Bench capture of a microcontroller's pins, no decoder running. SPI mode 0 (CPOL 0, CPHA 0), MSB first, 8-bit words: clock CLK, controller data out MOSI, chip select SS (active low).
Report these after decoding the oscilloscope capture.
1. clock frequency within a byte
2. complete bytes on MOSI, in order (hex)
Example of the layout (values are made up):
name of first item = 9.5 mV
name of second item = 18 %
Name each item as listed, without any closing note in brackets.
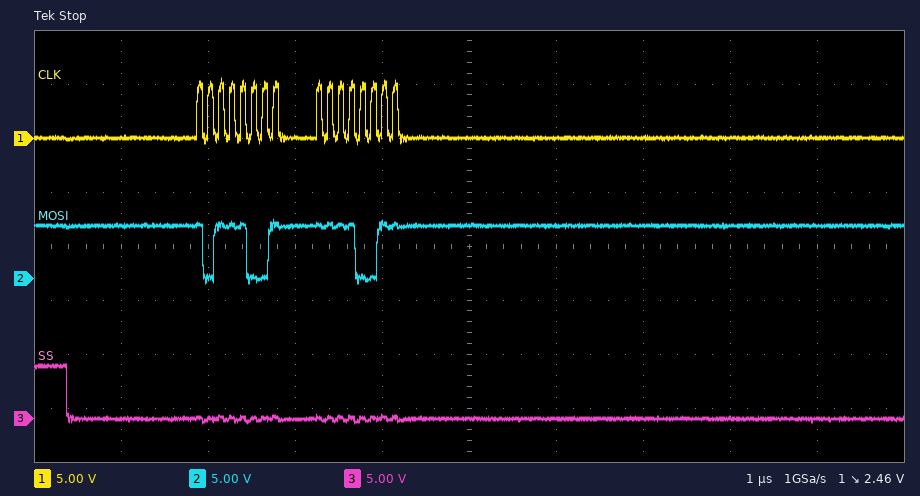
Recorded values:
clock frequency within a byte = 8 MHz
complete bytes on MOSI, in order = B9 F3
